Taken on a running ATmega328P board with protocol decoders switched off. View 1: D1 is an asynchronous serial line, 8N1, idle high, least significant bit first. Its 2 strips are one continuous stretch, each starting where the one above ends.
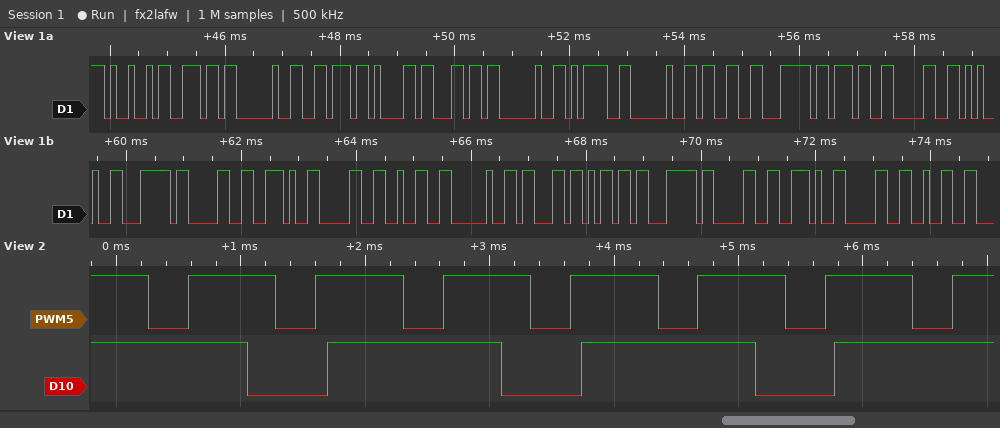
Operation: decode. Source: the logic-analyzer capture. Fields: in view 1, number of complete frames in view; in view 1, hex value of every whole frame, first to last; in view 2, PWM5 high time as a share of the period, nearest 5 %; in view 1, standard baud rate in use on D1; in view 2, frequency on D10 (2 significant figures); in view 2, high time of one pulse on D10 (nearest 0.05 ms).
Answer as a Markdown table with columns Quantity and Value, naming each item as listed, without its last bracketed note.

| Quantity | Value |
|---|---|
| in view 1, number of complete frames in view | 27 |
| in view 1, hex value of every whole frame, first to last | 49 6E 20 76 61 6C 20 3D 20 33 7C 37 30 25 7C 30 2E 30 32 20 63 6D 7C 30 2E 30 32 |
| in view 2, PWM5 high time as a share of the period, nearest 5 % | 70 % |
| in view 1, standard baud rate in use on D1 | 9600 baud |
| in view 2, frequency on D10 | 490 Hz |
| in view 2, high time of one pulse on D10 | 1.40 ms |
